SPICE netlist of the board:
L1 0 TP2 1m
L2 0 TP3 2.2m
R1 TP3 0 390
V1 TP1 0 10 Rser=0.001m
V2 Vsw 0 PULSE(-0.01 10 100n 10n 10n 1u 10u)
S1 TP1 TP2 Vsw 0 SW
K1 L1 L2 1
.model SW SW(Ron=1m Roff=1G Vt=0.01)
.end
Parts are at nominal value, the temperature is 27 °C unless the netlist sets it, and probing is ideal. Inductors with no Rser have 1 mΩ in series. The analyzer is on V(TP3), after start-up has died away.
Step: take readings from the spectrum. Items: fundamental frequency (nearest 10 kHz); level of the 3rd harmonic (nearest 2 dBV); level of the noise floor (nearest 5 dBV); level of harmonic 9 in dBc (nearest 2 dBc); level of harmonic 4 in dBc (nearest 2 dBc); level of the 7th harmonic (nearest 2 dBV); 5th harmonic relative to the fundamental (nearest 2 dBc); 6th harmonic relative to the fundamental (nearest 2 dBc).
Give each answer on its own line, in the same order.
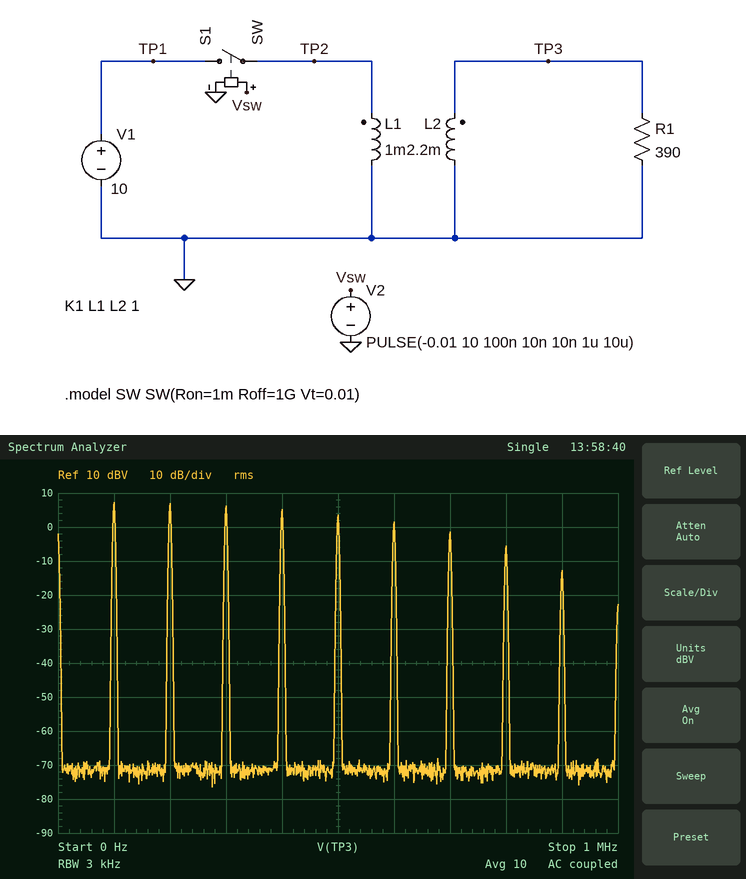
100 kHz
6 dBV
-70 dBV
-20 dBc
-2 dBc
-2 dBV
-4 dBc
-6 dBc
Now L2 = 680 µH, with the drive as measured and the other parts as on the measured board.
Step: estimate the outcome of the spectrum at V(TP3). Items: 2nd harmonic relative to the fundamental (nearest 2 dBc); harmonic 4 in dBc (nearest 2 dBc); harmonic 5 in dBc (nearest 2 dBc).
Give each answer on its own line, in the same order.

2 dBc
0 dBc
-2 dBc
